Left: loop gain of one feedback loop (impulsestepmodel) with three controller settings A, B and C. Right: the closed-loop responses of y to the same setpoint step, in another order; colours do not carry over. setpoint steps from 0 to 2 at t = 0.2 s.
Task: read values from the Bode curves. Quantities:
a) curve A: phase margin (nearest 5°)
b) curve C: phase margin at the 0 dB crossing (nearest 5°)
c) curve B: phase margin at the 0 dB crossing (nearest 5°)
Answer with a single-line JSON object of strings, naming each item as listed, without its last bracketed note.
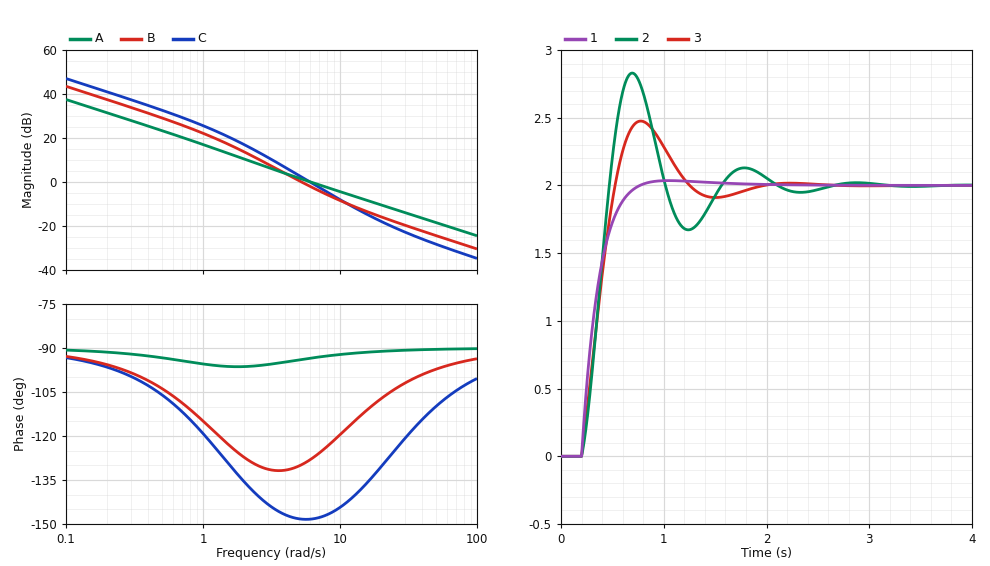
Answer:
{"curve A: phase margin": "85°", "curve C: phase margin at the 0 dB crossing": "30°", "curve B: phase margin at the 0 dB crossing": "50°"}
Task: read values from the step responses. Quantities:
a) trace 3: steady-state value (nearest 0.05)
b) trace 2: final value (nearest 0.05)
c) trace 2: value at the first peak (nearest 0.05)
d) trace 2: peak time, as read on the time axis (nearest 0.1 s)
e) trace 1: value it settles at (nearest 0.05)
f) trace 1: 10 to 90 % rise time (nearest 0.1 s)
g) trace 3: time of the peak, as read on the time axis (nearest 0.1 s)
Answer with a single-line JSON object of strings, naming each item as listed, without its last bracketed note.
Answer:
{"trace 3: steady-state value": "2.00", "trace 2: final value": "2.00", "trace 2: value at the first peak": "2.85", "trace 2: peak time, as read on the time axis": "0.7 s", "trace 1: value it settles at": "2.00", "trace 1: 10 to 90 % rise time": "0.3 s", "trace 3: time of the peak, as read on the time axis": "0.8 s"}
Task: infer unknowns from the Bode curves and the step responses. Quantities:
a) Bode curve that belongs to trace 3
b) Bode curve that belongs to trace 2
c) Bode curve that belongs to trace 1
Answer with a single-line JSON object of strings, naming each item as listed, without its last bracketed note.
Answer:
{"Bode curve that belongs to trace 3": "B", "Bode curve that belongs to trace 2": "C", "Bode curve that belongs to trace 1": "A"}
